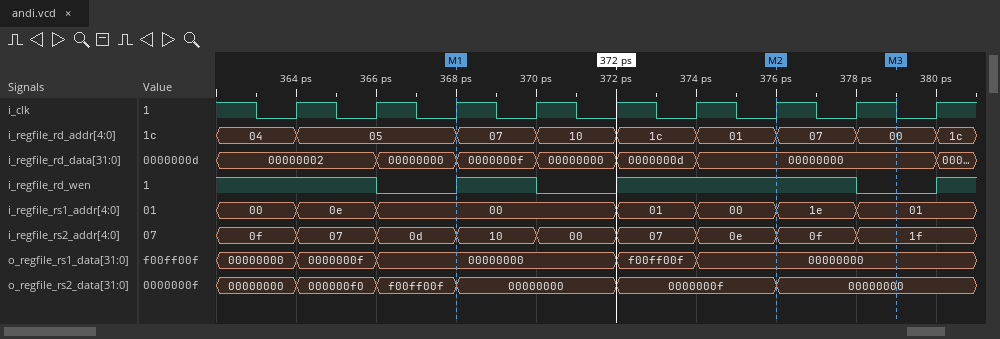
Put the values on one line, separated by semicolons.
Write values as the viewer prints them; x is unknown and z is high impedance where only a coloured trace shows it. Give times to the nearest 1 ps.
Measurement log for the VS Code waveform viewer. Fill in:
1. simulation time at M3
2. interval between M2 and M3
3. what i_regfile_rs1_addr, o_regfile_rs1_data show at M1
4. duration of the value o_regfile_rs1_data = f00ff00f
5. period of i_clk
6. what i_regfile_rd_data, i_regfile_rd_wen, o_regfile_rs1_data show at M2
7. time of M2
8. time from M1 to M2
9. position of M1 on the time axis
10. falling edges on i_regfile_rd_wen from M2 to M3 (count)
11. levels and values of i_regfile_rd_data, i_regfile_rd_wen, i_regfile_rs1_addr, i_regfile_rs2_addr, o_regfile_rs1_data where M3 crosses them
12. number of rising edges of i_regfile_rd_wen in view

379 ps; 3 ps; i_regfile_rs1_addr=00, o_regfile_rs1_data=00000000; 2 ps; 2 ps; i_regfile_rd_data=00000000, i_regfile_rd_wen=1, o_regfile_rs1_data=00000000; 376 ps; 8 ps; 368 ps; 1; i_regfile_rd_data=00000000, i_regfile_rd_wen=0, i_regfile_rs1_addr=01, i_regfile_rs2_addr=1f, o_regfile_rs1_data=00000000; 3
